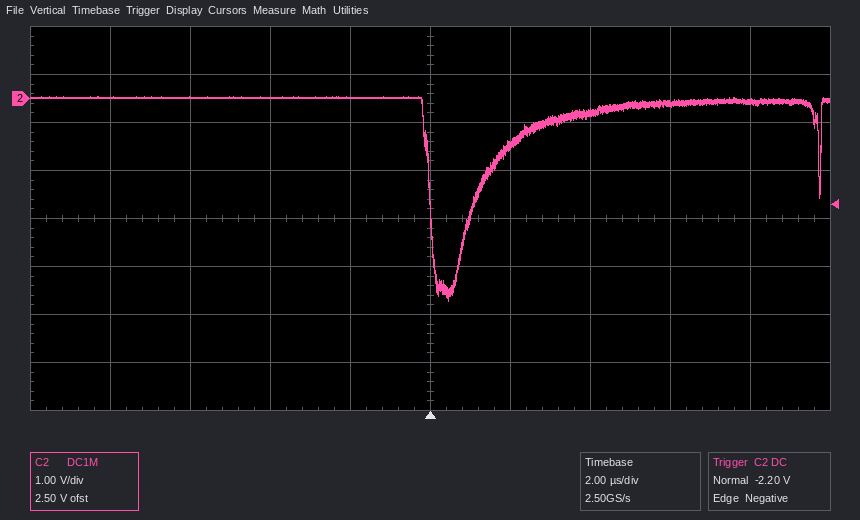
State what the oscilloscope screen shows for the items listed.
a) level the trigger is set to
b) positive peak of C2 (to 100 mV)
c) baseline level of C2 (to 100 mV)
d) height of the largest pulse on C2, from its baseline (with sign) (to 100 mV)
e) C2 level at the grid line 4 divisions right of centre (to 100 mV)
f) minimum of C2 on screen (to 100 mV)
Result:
-2.20 V
0.0 V
0.0 V
-4.2 V
-100 mV
-4.2 V
